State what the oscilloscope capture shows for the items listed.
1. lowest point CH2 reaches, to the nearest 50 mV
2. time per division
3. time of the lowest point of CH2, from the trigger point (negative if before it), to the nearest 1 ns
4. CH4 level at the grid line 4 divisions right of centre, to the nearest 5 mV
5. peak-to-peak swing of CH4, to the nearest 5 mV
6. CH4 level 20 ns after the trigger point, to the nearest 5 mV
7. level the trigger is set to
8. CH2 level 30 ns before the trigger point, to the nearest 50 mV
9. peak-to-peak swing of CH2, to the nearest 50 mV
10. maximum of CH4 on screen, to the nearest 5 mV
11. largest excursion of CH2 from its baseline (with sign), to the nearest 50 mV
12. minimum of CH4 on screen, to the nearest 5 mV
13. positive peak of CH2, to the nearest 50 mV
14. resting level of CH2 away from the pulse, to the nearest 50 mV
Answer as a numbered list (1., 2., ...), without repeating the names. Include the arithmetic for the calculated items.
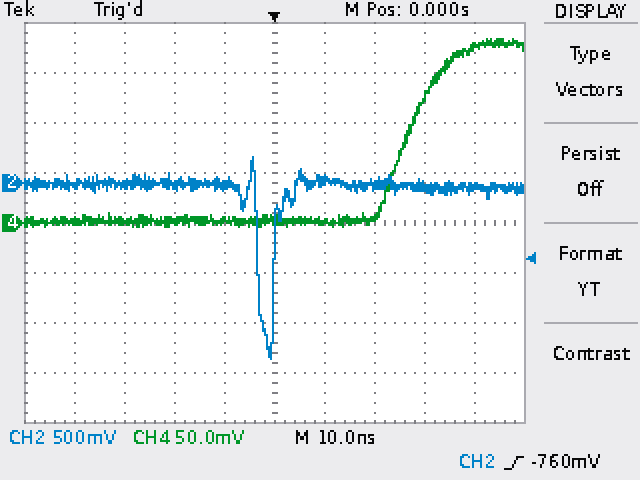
1. -1.75 V
2. 10 ns
3. -1 ns
4. 175 mV
5. 185 mV − (-5 mV) = 190 mV
6. 5 mV
7. -760 mV
8. 0 mV
9. 250 mV − (-1.75 V) = 2.00 V
10. 185 mV
11. -1.75 V − (0 mV) = -1.75 V
12. -5 mV
13. 250 mV
14. 0 mV
